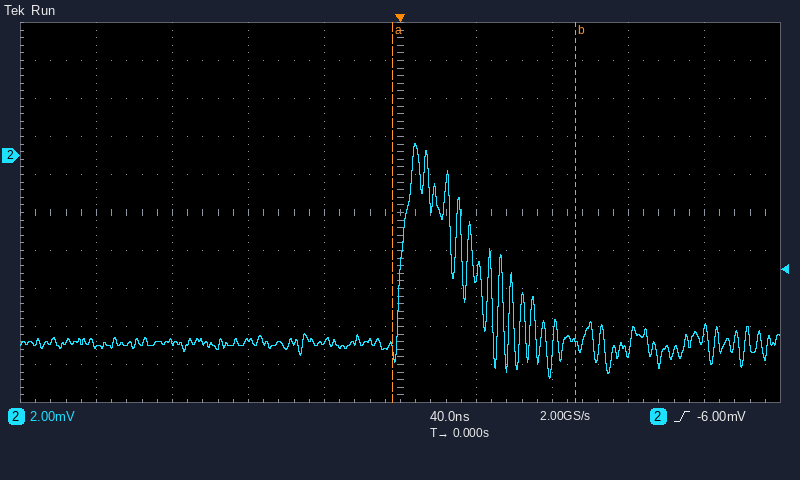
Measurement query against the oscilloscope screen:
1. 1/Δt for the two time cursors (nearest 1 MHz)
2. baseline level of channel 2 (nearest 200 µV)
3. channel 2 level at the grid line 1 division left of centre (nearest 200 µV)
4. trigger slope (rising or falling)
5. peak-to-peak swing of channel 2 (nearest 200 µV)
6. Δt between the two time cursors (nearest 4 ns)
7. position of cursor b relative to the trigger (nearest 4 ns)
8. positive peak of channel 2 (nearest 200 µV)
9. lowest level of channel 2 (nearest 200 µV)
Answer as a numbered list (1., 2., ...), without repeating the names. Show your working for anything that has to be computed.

1. 1 / 96 ns ≈ 10 MHz
2. -9.8 mV
3. -9.8 mV
4. rising
5. 600 µV − (-11.8 mV) = 12.4 mV
6. 96 ns
7. +92 ns
8. 600 µV
9. -11.8 mV
